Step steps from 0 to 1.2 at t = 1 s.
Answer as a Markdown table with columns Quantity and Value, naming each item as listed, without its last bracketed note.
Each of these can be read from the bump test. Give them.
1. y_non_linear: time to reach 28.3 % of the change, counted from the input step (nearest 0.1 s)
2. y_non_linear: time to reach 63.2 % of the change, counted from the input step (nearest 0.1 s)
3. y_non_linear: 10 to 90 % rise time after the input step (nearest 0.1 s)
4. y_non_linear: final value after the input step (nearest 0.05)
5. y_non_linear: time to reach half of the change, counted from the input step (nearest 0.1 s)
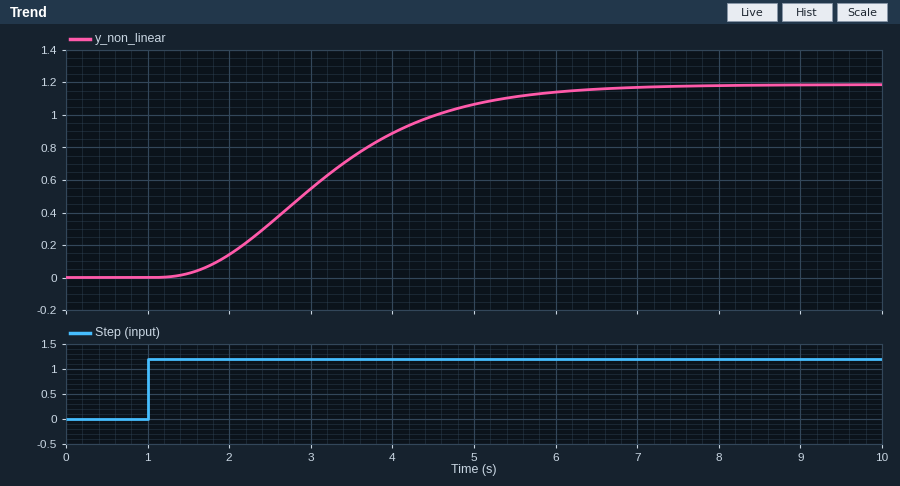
| Quantity | Value |
|---|---|
| y_non_linear: time to reach 28.3 % of the change, counted from the input step | 1.5 s |
| y_non_linear: time to reach 63.2 % of the change, counted from the input step | 2.5 s |
| y_non_linear: 10 to 90 % rise time after the input step | 3.1 s |
| y_non_linear: final value after the input step | 1.20 |
| y_non_linear: time to reach half of the change, counted from the input step | 2.1 s |
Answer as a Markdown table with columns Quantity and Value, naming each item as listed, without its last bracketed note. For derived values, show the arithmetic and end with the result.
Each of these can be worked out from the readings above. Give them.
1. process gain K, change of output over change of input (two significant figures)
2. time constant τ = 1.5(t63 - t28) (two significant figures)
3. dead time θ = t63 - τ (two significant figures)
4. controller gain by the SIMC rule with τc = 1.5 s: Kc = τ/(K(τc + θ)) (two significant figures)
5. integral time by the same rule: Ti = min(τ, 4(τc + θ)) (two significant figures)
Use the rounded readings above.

| Quantity | Value |
|---|---|
| process gain K, change of output over change of input | (1.2 - 0) / 1.2 = 1.0 |
| time constant τ = 1.5(t63 - t28) | 1.5 × (2.5 - 1.5) = 1.5 s |
| dead time θ = t63 - τ | 2.5 - 1.5 = 1.0 s |
| controller gain by the SIMC rule with τc = 1.5 s: Kc = τ/(K(τc + θ)) | 1.5 / (1 × (1.5 + 1)) = 0.60 |
| integral time by the same rule: Ti = min(τ, 4(τc + θ)) | min(1.5, 4 × (1.5 + 1)) = 1.5 s |
